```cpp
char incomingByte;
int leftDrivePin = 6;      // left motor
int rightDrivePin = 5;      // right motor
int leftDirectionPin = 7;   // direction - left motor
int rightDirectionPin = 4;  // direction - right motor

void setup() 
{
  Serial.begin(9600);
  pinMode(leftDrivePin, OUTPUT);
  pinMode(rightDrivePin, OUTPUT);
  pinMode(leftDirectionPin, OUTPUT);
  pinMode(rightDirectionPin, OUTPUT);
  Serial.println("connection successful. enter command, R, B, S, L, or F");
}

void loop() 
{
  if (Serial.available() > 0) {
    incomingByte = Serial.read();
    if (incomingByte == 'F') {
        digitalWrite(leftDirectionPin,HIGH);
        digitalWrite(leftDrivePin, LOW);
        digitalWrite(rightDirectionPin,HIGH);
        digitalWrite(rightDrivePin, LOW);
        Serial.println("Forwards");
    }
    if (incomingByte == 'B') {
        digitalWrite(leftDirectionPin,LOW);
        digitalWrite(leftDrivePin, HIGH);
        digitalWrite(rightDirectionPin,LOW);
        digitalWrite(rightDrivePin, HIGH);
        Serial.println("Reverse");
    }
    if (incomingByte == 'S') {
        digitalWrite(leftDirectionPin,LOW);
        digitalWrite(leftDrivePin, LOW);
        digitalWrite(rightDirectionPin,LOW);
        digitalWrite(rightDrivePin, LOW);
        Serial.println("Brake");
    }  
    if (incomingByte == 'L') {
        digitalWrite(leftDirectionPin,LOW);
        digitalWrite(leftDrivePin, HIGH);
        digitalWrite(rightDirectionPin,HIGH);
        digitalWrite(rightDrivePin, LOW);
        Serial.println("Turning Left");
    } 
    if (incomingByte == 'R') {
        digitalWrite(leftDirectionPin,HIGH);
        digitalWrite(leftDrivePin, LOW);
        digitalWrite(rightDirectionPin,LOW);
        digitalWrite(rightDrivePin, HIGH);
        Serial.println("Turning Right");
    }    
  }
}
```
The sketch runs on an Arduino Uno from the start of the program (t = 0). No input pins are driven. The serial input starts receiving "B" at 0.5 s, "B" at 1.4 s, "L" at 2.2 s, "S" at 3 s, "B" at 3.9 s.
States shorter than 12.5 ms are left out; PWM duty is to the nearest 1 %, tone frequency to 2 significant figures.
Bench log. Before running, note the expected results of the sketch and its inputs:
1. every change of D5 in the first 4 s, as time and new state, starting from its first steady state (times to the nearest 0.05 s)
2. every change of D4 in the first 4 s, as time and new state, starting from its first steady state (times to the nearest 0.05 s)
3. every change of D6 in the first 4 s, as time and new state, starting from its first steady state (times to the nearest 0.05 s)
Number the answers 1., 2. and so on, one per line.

1. 0 s low; 0.5 s high; 2.2 s low; 3.9 s high
2. 0 s low; 2.2 s high; 3 s low
3. 0 s low; 0.5 s high; 3 s low; 3.9 s high
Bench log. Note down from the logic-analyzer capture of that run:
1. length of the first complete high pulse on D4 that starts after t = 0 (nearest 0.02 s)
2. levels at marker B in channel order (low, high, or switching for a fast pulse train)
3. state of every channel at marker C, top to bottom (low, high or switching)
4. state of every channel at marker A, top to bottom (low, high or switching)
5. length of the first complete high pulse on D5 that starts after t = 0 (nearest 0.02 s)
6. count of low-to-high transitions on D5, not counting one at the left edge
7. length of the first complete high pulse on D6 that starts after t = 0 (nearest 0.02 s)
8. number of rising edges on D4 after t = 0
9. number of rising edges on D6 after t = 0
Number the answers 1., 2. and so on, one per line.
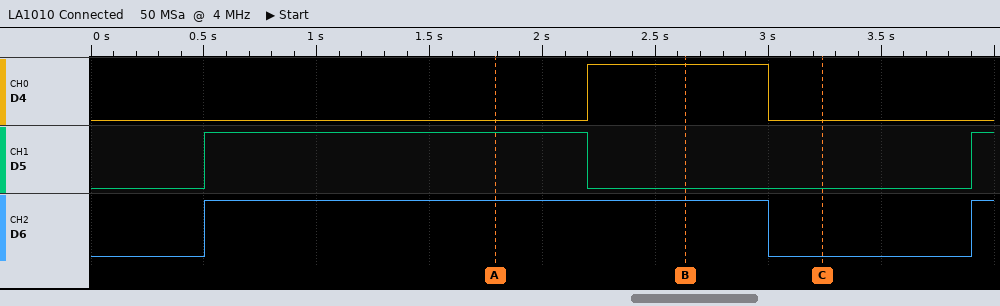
1. 0.80 s
2. D4 high, D5 low, D6 high
3. D4 low, D5 low, D6 low
4. D4 low, D5 high, D6 high
5. 1.70 s
6. 2
7. 2.50 s
8. 1
9. 2
